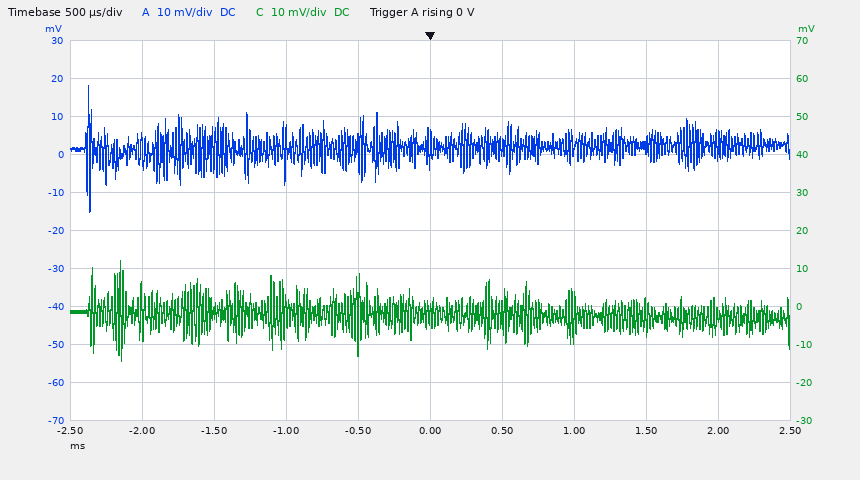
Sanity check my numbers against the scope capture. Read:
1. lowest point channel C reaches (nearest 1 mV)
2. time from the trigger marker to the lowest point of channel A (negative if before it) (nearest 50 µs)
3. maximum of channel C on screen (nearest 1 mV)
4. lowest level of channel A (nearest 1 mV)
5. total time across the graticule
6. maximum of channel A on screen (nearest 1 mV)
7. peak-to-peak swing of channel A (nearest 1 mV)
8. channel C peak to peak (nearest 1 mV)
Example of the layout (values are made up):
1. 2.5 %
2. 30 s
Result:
1. -14 mV
2. -2.35 ms
3. 12 mV
4. -15 mV
5. 5 ms
6. 18 mV
7. 33 mV
8. 26 mV
